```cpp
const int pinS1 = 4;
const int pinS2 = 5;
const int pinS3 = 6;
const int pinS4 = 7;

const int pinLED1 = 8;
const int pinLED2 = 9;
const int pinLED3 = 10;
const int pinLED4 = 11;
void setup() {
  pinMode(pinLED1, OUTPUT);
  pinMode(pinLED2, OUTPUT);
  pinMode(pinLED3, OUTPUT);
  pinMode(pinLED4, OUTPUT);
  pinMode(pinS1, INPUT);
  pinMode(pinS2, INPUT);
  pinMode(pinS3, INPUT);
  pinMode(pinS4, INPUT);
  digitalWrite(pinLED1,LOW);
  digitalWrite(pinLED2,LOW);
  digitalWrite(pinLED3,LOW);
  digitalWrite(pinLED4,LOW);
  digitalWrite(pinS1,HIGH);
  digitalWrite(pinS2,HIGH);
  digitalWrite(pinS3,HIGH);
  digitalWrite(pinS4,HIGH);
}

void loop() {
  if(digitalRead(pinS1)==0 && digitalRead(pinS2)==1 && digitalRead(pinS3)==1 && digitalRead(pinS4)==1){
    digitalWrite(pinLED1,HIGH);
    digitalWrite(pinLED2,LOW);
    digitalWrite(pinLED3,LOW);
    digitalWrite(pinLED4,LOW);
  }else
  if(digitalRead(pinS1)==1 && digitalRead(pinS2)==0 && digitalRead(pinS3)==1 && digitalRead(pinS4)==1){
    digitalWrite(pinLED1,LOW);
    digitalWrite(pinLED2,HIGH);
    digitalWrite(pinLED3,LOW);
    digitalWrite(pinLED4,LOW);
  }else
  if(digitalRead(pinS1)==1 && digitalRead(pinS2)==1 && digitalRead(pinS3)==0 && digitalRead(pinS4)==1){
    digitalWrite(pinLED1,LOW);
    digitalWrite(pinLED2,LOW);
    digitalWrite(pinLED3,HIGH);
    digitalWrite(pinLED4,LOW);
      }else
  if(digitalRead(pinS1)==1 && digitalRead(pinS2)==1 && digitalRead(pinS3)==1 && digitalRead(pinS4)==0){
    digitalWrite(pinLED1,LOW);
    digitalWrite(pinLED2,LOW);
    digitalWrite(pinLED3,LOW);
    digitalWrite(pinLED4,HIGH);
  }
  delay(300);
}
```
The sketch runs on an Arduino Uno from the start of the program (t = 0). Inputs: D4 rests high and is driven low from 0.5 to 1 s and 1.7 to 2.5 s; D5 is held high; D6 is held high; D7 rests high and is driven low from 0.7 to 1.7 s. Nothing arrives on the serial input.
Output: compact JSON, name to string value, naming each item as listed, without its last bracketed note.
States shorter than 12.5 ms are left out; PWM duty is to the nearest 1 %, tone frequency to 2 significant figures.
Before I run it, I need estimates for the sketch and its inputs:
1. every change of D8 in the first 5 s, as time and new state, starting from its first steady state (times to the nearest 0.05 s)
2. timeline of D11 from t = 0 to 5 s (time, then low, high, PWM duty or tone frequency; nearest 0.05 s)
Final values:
{"every change of D8 in the first 5 s, as time and new state, starting from its first steady state": "0 s low; 0.6 s high; 1.2 s low; 1.8 s high", "timeline of D11 from t = 0 to 5 s": "0 s low; 1.2 s high; 1.8 s low"}
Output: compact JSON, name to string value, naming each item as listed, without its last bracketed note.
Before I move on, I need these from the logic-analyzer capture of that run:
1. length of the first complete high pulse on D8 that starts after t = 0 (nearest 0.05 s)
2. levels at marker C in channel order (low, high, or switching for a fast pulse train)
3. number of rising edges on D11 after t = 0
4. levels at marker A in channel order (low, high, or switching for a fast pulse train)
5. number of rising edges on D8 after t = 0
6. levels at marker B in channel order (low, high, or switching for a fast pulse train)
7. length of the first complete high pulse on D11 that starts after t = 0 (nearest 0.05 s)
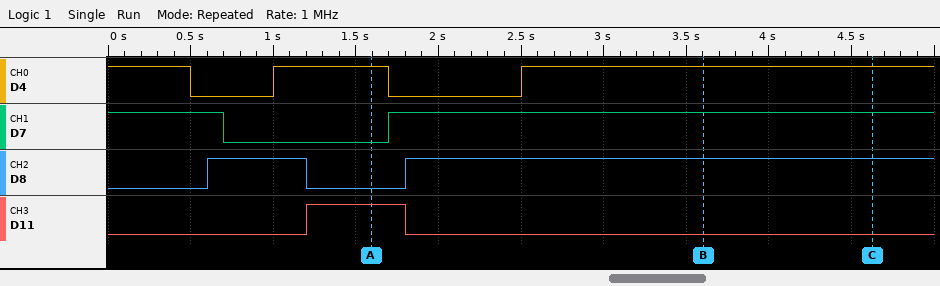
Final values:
{"length of the first complete high pulse on D8 that starts after t = 0": "0.60 s", "levels at marker C in channel order": "D4 high, D7 high, D8 high, D11 low", "number of rising edges on D11 after t = 0": "1", "levels at marker A in channel order": "D4 high, D7 low, D8 low, D11 high", "number of rising edges on D8 after t = 0": "2", "levels at marker B in channel order": "D4 high, D7 high, D8 high, D11 low", "length of the first complete high pulse on D11 that starts after t = 0": "0.60 s"}
